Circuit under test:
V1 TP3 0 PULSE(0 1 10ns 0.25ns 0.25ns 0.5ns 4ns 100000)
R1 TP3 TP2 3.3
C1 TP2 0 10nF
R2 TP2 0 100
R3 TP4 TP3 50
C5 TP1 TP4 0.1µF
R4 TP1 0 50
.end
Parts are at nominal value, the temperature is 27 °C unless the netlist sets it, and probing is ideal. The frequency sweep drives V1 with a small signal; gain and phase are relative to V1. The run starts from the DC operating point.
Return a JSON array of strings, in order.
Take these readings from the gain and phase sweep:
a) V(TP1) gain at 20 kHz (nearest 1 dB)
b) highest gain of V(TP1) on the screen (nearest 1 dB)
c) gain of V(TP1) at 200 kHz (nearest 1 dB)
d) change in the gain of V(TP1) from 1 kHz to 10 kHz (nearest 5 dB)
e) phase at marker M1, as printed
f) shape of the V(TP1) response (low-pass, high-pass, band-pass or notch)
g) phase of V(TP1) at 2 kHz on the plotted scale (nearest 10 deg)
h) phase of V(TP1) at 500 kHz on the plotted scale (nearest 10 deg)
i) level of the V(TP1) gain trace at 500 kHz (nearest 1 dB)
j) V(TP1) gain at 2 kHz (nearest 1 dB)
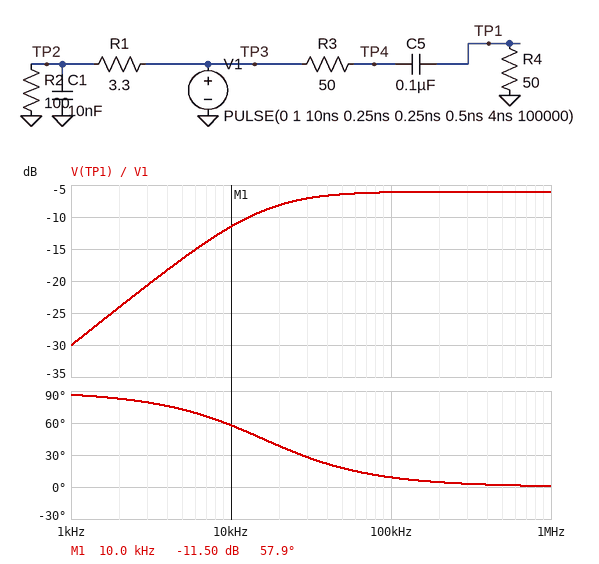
["-8 dB", "-6 dB", "-6 dB", "20 dB", "57.9 deg", "high-pass", "80 deg", "0 deg", "-6 dB", "-24 dB"]
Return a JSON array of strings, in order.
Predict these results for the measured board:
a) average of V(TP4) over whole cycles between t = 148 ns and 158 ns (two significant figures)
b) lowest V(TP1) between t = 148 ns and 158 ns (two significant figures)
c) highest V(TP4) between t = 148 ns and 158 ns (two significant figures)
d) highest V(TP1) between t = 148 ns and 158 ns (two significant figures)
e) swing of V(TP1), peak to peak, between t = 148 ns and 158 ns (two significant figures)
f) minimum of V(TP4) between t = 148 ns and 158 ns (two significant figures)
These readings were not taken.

["95 mV", "-1.4 mV", "500 mV", "500 mV", "500 mV", "1.3 mV"]
